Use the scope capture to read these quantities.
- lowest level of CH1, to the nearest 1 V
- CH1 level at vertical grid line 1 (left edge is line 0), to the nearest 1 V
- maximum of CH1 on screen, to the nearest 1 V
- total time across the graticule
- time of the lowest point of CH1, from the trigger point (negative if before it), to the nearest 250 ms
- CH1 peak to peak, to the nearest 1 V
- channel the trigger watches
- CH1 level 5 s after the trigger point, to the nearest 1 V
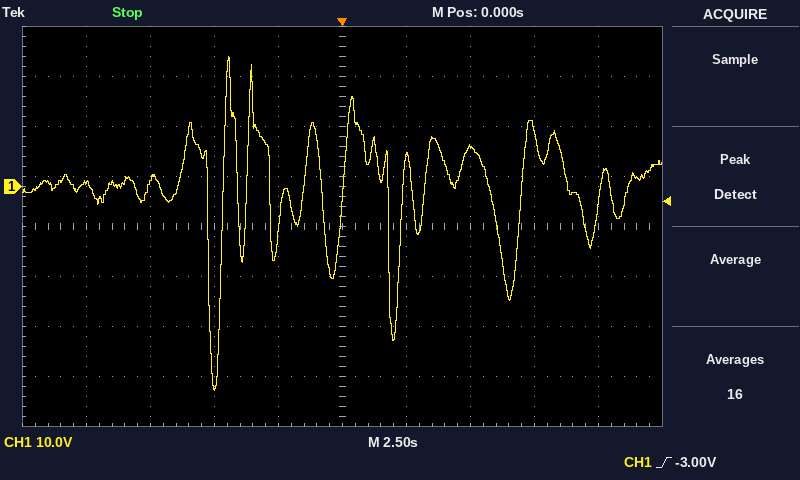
-41 V
1 V
26 V
25 s
-5.00 s
67 V
CH1
8 V
